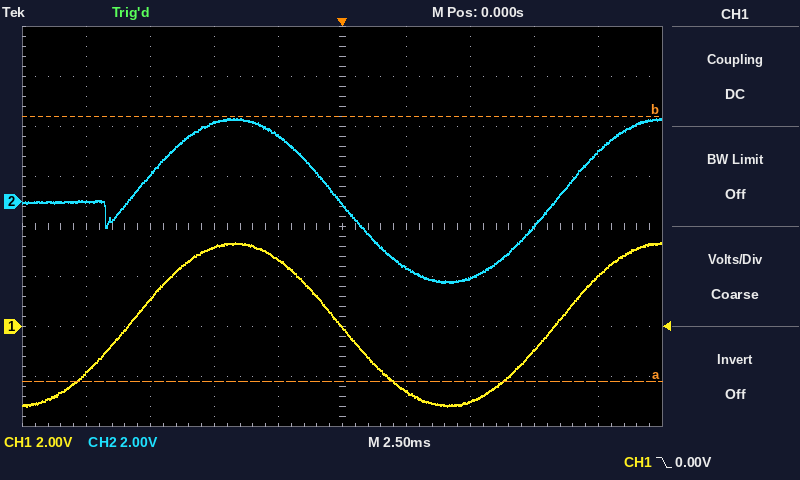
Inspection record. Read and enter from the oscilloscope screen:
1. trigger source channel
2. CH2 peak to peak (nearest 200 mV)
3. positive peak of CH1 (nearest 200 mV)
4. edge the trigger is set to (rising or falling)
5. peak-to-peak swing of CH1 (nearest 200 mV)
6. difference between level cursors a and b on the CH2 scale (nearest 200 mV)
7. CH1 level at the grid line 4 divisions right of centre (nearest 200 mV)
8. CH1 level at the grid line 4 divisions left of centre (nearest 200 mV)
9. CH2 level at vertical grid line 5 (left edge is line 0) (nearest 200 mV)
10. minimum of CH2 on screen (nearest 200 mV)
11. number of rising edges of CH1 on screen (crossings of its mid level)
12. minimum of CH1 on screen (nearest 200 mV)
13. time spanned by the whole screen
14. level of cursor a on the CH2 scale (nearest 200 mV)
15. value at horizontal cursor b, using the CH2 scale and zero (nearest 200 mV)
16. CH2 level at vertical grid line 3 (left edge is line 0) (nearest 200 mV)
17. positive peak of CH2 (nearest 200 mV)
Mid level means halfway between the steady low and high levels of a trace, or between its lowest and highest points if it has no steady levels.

CH1
6.6 V
3.4 V
falling
6.6 V
10.6 V
2.0 V
-1.8 V
0.0 V
-3.2 V
2
-3.2 V
25 ms
-7.2 V
3.4 V
3.2 V
3.4 V
